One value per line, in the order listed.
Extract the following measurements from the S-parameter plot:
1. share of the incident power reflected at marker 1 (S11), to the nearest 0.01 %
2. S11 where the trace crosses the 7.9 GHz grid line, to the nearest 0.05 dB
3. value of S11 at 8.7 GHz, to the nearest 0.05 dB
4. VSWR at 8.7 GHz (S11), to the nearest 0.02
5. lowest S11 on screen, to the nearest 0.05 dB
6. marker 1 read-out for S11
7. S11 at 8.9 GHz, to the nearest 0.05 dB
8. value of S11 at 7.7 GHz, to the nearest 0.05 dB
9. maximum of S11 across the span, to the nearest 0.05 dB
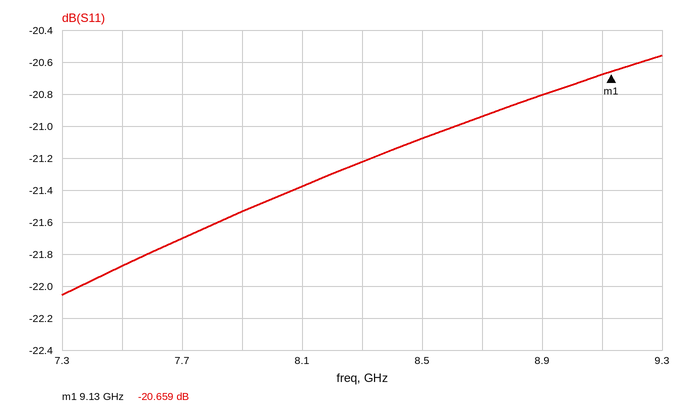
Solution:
0.86 %
-21.55 dB
-20.95 dB
1.20
-22.05 dB
-20.659 dB
-20.80 dB
-21.70 dB
-20.55 dB
